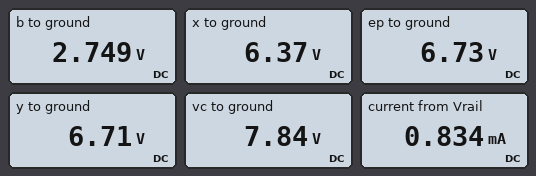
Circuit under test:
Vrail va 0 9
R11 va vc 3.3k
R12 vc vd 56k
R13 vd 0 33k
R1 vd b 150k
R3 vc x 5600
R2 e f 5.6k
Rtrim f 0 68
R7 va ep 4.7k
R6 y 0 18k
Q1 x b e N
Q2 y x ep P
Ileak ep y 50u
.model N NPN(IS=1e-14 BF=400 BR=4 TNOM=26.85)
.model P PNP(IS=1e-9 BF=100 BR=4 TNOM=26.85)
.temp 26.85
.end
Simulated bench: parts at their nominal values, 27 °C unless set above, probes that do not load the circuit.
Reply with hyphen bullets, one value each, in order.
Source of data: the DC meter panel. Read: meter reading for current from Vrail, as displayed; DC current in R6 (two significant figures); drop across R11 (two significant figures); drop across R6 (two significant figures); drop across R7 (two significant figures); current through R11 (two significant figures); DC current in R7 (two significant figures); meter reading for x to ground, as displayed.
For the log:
- 0.834 mA
- 370 µA
- 1.2 V
- 6.7 V
- 2.3 V
- 350 µA
- 480 µA
- 6.37 V
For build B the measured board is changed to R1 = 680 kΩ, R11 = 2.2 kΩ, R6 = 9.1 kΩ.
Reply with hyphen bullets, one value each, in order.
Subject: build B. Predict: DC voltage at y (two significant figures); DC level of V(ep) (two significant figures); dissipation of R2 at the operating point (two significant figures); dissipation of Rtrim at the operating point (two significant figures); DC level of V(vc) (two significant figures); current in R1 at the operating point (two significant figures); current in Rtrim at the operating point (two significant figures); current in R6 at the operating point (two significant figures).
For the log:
- 4.5 V
- 6.7 V
- 580 µW
- 7.0 µW
- 8.1 V
- 800 nA
- 320 µA
- 490 µA
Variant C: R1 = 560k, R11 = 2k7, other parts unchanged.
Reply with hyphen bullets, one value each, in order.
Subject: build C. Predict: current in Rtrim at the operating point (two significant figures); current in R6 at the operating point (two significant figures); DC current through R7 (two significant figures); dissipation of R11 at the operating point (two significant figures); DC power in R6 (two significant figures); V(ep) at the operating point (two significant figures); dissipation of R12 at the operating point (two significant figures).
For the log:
- 330 µA
- 380 µA
- 450 µA
- 340 µW
- 2.6 mW
- 6.9 V
- 460 µW
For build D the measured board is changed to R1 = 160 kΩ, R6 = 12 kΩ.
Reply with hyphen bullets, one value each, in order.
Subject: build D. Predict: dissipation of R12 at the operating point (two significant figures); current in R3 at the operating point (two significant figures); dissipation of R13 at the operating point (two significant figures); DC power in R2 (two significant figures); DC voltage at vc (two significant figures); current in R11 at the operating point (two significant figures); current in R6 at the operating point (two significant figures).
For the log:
- 420 µW
- 310 µA
- 240 µW
- 740 µW
- 7.7 V
- 400 µA
- 520 µA
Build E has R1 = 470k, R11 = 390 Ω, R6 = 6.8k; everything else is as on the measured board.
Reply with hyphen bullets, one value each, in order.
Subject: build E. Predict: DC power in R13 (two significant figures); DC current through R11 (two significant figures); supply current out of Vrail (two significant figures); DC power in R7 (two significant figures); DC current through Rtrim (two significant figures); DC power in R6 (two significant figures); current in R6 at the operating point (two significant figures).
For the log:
- 320 µW
- 480 µA
- 900 µA
- 830 µW
- 380 µA
- 1.2 mW
- 420 µA
